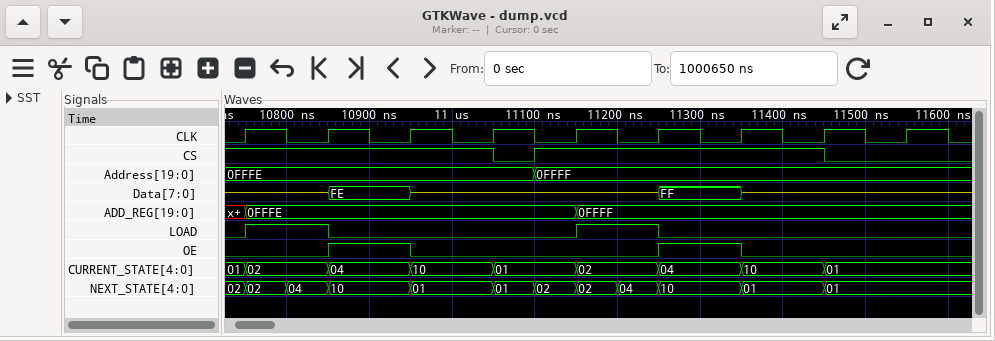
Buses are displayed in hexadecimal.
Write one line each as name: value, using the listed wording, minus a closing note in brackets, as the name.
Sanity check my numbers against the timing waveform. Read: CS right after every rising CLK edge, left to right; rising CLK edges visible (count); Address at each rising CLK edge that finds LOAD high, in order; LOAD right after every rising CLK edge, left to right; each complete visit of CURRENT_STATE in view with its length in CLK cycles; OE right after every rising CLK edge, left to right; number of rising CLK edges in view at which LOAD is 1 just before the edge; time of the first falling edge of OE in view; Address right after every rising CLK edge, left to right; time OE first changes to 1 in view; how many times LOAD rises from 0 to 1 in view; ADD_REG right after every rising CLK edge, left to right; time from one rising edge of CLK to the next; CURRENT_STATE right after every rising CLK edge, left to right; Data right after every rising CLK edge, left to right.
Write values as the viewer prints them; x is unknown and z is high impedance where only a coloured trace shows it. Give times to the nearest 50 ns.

CS right after every rising CLK edge, left to right: 1 1 1 0 1 1 1 0 0
rising CLK edges visible: 9
Address at each rising CLK edge that finds LOAD high, in order: 0FFFE, 0FFFF
LOAD right after every rising CLK edge, left to right: 1 0 0 0 1 0 0 0 0
each complete visit of CURRENT_STATE in view with its length in CLK cycles: 02: 1, 04: 1, 10: 1, 01: 1, 02: 1, 04: 1, 10: 1
OE right after every rising CLK edge, left to right: 0 1 0 0 0 1 0 0 0
number of rising CLK edges in view at which LOAD is 1 just before the edge: 2
time of the first falling edge of OE in view: 10950 ns
Address right after every rising CLK edge, left to right: 0FFFE, 0FFFE, 0FFFE, 0FFFE, 0FFFF, 0FFFF, 0FFFF, 0FFFF, 0FFFF
time OE first changes to 1 in view: 10850 ns
how many times LOAD rises from 0 to 1 in view: 2
ADD_REG right after every rising CLK edge, left to right: 0FFFE, 0FFFE, 0FFFE, 0FFFE, 0FFFF, 0FFFF, 0FFFF, 0FFFF, 0FFFF
time from one rising edge of CLK to the next: 100 ns
CURRENT_STATE right after every rising CLK edge, left to right: 02, 04, 10, 01, 02, 04, 10, 01, 01
Data right after every rising CLK edge, left to right: z, FE, z, z, z, FF, z, z, z
